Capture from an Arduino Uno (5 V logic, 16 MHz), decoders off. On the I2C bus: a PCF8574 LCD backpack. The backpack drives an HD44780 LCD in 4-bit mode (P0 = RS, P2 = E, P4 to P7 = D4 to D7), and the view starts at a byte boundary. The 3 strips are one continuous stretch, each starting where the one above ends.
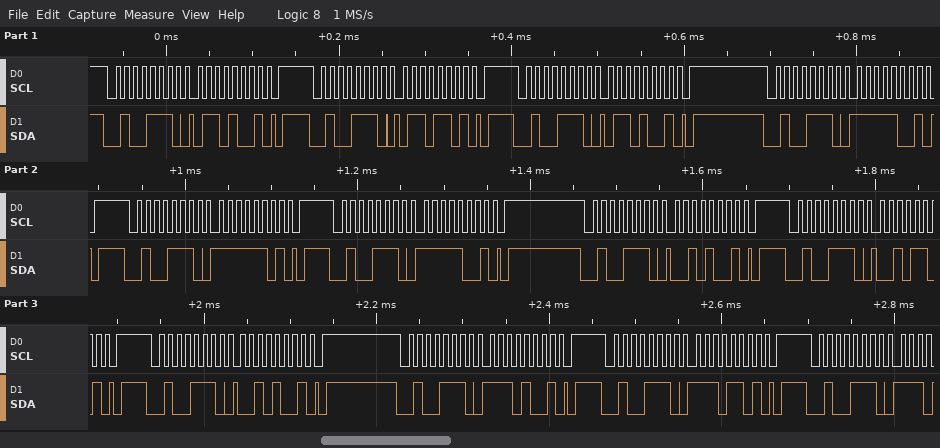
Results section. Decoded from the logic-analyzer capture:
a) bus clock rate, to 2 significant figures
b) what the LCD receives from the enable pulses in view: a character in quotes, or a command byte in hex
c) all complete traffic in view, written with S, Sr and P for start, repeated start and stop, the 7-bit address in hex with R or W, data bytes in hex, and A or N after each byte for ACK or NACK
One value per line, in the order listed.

100 kHz
'o'
S 27W A 69 A P S 27W A 6D A P S 27W A 69 A P S 27W A F9 A P S 27W A FD A P S 27W A F9 A P S 27W A 29 A P S 27W A 2D A P S 27W A 29 A P S 27W A E9 A P S 27W A ED A P S 27W A
